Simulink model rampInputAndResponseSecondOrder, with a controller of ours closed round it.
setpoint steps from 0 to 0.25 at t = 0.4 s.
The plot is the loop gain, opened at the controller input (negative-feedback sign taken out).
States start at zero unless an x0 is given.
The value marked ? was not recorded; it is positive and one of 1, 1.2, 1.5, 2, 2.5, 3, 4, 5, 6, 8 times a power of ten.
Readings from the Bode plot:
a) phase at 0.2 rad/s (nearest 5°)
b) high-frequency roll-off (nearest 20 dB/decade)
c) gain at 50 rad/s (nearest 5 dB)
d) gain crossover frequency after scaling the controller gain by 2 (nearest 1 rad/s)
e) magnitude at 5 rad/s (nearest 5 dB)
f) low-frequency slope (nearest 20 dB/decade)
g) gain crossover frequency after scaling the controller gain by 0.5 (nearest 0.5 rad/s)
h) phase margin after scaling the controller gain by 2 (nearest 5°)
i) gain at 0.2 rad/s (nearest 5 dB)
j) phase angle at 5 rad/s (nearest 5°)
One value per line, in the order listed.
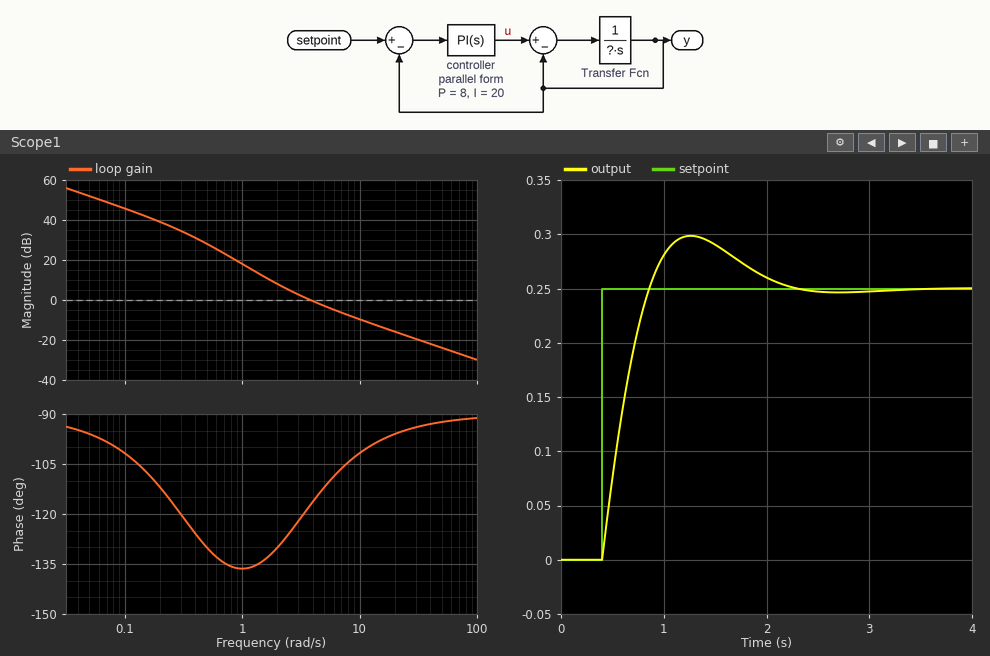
-110°
-20 dB/decade
-25 dB
7 rad/s
-5 dB
-20 dB/decade
2.5 rad/s
75°
40 dB
-110°
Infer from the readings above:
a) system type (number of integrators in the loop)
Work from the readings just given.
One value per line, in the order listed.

1
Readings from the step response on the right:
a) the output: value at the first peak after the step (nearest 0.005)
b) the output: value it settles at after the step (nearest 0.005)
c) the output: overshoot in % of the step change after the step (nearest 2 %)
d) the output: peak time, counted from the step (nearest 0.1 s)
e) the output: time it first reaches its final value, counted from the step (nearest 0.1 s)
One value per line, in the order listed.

0.300
0.250
20 %
0.9 s
0.5 s
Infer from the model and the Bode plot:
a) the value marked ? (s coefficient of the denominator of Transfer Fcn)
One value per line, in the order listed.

2.5
